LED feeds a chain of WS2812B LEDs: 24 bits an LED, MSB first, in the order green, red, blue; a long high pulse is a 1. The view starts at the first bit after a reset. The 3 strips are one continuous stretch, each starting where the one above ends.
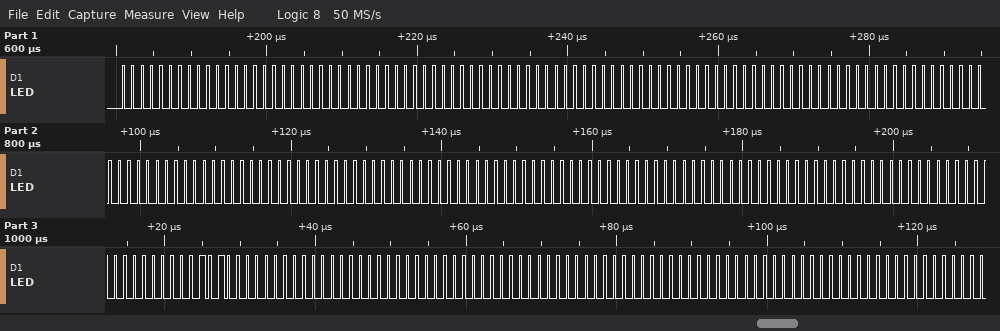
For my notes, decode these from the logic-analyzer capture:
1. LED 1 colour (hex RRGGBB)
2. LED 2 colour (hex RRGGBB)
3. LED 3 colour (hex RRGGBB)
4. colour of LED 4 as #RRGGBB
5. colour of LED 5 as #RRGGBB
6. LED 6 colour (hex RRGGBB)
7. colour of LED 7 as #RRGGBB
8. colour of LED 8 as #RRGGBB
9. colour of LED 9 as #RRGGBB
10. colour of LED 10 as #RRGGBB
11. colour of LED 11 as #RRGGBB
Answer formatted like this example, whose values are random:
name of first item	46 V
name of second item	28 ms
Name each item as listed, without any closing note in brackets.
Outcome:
LED 1 colour	#000000
LED 2 colour	#000000
LED 3 colour	#000000
colour of LED 4 as #RRGGBB	#000000
colour of LED 5 as #RRGGBB	#000000
LED 6 colour	#000000
colour of LED 7 as #RRGGBB	#000000
colour of LED 8 as #RRGGBB	#000000
colour of LED 9 as #RRGGBB	#001400
colour of LED 10 as #RRGGBB	#000000
colour of LED 11 as #RRGGBB	#000000
